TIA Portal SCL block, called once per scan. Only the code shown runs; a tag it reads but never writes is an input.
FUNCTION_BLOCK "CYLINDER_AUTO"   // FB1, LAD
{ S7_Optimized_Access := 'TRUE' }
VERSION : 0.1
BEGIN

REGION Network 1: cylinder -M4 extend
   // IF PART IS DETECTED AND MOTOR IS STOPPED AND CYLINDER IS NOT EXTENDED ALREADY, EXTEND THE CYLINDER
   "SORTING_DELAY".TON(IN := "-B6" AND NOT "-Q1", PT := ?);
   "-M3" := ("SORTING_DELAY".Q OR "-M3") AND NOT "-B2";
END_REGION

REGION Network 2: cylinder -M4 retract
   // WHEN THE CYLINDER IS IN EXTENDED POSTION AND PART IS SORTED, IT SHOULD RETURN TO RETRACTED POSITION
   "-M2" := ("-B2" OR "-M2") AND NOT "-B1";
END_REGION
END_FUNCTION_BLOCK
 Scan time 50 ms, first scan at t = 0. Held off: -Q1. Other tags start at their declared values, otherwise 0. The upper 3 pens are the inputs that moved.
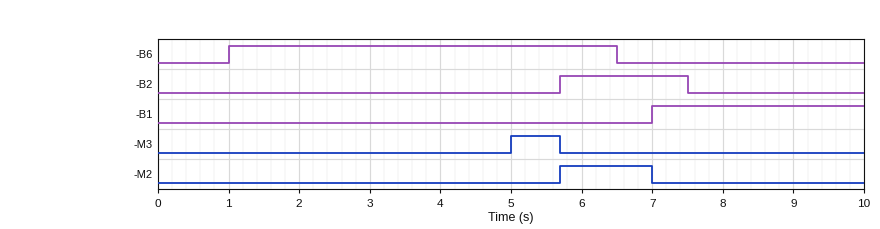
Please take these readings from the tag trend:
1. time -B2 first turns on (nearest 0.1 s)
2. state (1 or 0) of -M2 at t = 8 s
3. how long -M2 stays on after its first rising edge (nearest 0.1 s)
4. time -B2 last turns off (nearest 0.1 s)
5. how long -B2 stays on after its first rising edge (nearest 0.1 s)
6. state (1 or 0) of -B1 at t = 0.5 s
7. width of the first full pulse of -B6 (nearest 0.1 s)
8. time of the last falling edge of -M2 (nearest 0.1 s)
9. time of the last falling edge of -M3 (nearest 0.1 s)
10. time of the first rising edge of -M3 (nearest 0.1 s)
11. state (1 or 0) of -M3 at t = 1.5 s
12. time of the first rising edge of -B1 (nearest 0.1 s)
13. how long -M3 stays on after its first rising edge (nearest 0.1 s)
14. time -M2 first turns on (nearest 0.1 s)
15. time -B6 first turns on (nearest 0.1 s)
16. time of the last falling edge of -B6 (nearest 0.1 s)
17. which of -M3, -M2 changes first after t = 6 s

5.7 s
0
1.3 s
7.5 s
1.8 s
0
5.5 s
7.0 s
5.7 s
5.0 s
0
7.0 s
0.7 s
5.7 s
1.0 s
6.5 s
-M2
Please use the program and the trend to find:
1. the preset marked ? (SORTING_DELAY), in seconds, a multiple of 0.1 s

4.0 s
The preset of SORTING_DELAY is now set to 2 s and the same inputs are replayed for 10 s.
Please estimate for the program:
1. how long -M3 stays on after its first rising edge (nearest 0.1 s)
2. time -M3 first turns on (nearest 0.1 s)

2.7 s
3.0 s
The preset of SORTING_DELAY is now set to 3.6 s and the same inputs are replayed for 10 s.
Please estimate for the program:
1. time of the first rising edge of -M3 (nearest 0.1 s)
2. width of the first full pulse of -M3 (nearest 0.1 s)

4.6 s
1.1 s
